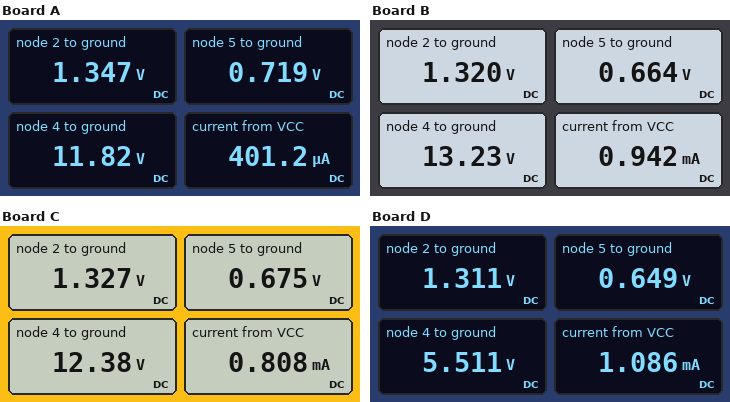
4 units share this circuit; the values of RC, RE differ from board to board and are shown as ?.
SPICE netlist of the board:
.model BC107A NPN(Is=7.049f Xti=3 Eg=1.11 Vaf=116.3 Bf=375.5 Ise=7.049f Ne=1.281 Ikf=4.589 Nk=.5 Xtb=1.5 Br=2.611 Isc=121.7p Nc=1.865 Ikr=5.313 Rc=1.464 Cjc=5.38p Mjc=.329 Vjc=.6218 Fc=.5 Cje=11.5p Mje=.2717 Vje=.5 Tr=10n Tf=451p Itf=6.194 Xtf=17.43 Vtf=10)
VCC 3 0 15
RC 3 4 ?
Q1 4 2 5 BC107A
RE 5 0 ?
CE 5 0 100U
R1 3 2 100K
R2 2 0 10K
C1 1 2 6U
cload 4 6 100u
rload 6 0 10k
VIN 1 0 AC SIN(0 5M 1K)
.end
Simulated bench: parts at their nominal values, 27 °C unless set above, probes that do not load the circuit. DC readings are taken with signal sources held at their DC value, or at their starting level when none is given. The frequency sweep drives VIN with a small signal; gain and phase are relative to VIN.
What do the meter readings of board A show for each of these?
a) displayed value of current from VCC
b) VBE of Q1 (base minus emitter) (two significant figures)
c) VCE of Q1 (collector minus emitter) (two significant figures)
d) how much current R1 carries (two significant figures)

401.2 µA
630 mV
11 V
140 µA
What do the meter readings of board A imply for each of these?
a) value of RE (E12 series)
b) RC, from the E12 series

2.7 kΩ
12 kΩ
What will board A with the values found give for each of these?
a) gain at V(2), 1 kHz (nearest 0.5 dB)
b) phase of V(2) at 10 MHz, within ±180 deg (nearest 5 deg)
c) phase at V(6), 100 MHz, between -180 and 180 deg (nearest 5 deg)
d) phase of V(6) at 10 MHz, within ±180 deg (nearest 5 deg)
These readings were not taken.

0 dB
0 deg
90 deg
145 deg
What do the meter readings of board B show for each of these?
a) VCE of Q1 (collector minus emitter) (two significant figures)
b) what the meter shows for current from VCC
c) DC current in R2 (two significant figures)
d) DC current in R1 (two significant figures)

13 V
0.942 mA
130 µA
140 µA
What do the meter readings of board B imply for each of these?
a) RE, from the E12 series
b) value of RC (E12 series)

820 Ω
2.2 kΩ
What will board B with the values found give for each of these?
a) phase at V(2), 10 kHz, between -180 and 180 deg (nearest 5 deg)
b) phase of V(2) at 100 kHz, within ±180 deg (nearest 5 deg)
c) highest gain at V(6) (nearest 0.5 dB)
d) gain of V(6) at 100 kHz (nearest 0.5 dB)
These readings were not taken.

0 deg
0 deg
35.0 dB
35.0 dB
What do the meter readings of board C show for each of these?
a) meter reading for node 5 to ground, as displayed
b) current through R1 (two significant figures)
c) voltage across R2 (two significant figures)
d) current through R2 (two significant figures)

0.675 V
140 µA
1.3 V
130 µA
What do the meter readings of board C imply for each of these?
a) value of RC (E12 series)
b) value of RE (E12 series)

3.9 kΩ
1 kΩ
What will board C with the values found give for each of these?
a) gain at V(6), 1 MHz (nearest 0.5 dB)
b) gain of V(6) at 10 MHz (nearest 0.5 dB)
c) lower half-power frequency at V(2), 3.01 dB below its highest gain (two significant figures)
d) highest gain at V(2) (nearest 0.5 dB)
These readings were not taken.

37.0 dB
36.5 dB
3.4 Hz
0 dB
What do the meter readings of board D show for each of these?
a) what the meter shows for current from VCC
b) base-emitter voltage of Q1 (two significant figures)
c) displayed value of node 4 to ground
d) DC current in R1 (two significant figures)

1.086 mA
660 mV
5.511 V
140 µA
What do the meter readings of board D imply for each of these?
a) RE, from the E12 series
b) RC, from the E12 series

680 Ω
10 kΩ
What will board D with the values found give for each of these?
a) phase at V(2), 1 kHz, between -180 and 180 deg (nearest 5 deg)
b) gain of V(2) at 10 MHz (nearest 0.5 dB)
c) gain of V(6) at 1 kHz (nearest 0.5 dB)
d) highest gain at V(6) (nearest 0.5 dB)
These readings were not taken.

0 deg
0 dB
45.0 dB
45.0 dB
